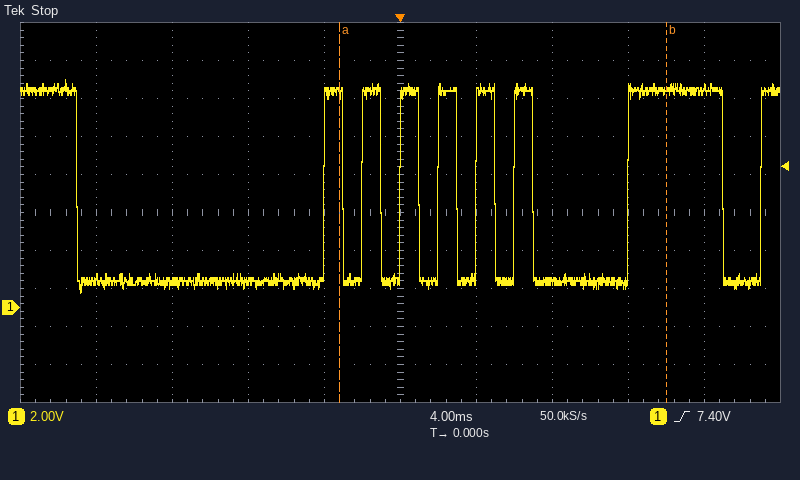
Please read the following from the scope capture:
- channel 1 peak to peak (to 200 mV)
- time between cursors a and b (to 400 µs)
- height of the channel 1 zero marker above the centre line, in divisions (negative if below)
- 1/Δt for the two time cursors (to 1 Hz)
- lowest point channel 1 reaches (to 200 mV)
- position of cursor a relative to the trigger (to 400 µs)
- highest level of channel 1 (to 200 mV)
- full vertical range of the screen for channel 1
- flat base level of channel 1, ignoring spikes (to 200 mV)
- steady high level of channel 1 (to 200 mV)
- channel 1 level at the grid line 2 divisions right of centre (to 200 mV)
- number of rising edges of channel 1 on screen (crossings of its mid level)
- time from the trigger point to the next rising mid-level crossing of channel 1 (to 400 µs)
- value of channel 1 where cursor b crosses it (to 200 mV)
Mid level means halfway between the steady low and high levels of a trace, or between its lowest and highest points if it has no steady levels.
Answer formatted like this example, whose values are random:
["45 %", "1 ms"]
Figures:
["11.2 V", "17.2 ms", "-2.5 div", "58 Hz", "800 mV", "-3.2 ms", "12.0 V", "20 V", "1.4 V", "11.4 V", "1.4 V", "8", "2.0 ms", "11.4 V"]
